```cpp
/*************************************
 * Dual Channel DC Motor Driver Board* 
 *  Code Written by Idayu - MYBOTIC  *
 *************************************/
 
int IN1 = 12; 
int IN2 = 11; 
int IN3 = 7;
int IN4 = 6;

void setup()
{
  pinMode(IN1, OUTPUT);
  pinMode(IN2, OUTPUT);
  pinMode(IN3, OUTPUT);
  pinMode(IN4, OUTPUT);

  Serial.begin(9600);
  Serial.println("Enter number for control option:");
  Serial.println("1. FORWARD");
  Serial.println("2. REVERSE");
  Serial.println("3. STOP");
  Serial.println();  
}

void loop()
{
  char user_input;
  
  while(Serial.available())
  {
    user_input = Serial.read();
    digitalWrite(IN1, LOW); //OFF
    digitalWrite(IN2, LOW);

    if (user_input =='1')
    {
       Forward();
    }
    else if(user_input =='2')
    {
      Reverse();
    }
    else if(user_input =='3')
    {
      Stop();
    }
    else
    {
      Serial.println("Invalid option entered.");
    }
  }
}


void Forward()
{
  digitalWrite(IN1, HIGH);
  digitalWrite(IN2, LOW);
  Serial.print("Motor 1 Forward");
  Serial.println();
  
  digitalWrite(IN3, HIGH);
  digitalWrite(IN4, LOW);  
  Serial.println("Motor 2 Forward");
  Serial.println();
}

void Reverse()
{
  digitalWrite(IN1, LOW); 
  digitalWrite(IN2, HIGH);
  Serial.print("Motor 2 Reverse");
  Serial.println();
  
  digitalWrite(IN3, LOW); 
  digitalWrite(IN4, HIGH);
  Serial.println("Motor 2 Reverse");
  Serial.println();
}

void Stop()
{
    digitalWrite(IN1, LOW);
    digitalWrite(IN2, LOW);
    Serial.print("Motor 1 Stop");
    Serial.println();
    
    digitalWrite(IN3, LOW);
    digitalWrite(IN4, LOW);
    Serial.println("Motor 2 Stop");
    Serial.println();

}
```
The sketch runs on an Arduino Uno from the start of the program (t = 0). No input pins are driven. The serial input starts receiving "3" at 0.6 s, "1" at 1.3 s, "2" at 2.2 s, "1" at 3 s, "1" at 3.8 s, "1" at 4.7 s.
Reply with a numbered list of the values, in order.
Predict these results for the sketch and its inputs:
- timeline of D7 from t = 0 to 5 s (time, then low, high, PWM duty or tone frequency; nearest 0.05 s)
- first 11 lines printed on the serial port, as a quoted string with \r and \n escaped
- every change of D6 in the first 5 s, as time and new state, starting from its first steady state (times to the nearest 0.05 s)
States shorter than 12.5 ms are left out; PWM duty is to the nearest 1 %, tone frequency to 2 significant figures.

1. 0 s low; 1.3 s high; 2.2 s low; 3 s high
2. "Enter number for control option:\r\n1. FORWARD\r\n2. REVERSE\r\n3. STOP\r\n\r\nMotor 1 Stop\r\nMotor 2 Stop\r\n\r\nMotor 1 Forward\r\nMotor 2 Forward\r\n\r\n"
3. 0 s low; 2.2 s high; 3 s low
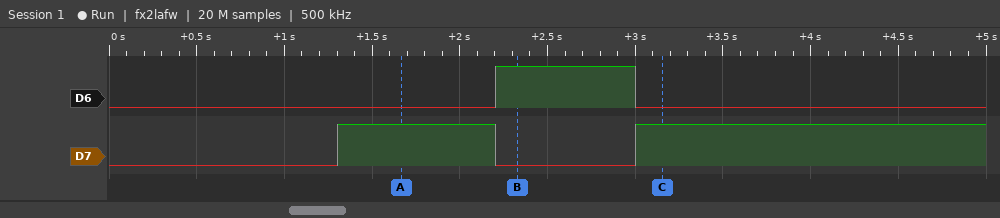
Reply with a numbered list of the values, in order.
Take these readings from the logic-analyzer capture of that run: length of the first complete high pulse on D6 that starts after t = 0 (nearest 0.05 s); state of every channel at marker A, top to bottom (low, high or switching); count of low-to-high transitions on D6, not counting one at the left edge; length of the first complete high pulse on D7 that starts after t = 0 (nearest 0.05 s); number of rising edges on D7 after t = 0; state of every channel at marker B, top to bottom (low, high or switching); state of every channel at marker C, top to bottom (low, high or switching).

1. 0.80 s
2. D6 low, D7 high
3. 1
4. 0.90 s
5. 2
6. D6 high, D7 low
7. D6 low, D7 high
